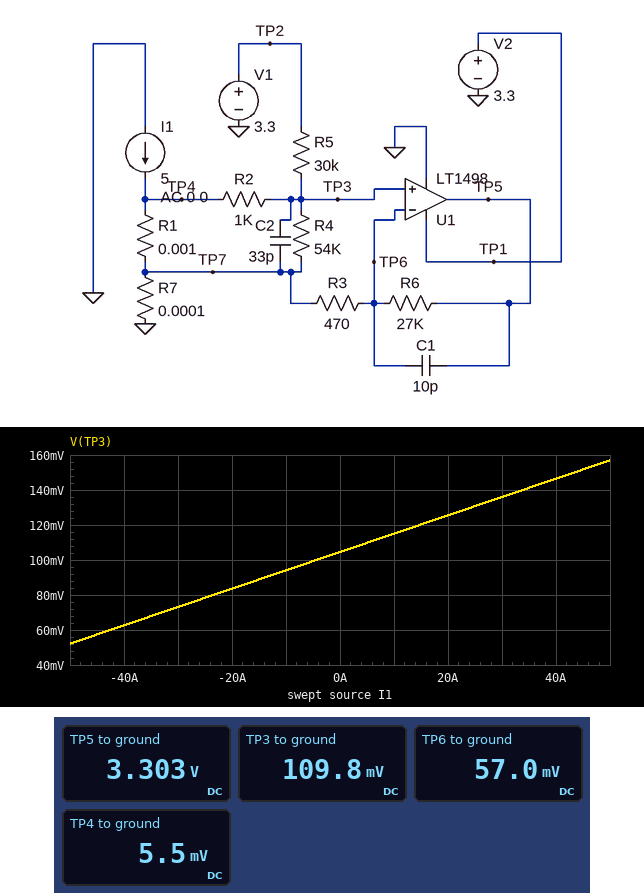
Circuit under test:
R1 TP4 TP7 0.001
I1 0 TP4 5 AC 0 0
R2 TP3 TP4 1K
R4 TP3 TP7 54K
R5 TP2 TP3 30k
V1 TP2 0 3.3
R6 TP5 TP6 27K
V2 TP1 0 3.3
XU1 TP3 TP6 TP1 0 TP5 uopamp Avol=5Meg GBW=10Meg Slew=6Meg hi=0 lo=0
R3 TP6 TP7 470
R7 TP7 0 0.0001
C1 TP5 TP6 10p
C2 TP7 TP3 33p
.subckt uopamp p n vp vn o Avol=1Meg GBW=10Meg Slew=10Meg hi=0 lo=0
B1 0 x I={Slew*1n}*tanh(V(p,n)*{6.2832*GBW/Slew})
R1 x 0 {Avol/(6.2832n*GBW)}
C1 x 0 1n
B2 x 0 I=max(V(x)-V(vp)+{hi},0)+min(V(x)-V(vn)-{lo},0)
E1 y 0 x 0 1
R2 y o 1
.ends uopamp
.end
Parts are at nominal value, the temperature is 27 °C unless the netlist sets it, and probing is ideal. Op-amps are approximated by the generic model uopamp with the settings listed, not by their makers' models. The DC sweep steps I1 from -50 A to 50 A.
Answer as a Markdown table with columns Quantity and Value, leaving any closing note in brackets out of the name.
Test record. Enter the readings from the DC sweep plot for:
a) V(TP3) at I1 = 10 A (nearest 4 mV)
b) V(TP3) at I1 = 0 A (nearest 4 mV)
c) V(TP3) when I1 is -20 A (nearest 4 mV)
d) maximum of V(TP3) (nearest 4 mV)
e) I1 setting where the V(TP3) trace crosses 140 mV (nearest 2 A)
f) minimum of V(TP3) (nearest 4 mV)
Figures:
| Quantity | Value |
|---|---|
| V(TP3) at I1 = 10 A | 116 mV |
| V(TP3) at I1 = 0 A | 104 mV |
| V(TP3) when I1 is -20 A | 84 mV |
| maximum of V(TP3) | 156 mV |
| I1 setting where the V(TP3) trace crosses 140 mV | 34 A |
| minimum of V(TP3) | 52 mV |
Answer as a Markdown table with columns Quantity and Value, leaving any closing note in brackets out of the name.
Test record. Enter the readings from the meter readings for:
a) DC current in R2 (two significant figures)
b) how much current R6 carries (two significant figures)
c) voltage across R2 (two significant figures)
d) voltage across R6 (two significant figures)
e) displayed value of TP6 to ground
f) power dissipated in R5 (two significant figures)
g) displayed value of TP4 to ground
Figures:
| Quantity | Value |
|---|---|
| DC current in R2 | 100 µA |
| how much current R6 carries | 120 µA |
| voltage across R2 | 100 mV |
| voltage across R6 | 3.2 V |
| displayed value of TP6 to ground | 57.0 mV |
| power dissipated in R5 | 340 µW |
| displayed value of TP4 to ground | 5.5 mV |
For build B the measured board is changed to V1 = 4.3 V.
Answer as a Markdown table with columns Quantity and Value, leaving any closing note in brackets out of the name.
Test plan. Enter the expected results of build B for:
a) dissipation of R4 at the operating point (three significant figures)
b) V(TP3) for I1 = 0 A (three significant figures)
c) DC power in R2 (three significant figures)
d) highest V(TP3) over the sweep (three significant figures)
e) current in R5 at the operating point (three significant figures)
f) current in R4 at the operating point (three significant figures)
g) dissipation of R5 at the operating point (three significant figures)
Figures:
| Quantity | Value |
|---|---|
| dissipation of R4 at the operating point | 368 nW |
| V(TP3) for I1 = 0 A | 136 mV |
| DC power in R2 | 18.5 µW |
| highest V(TP3) over the sweep | 189 mV |
| current in R5 at the operating point | 139 µA |
| current in R4 at the operating point | 2.61 µA |
| dissipation of R5 at the operating point | 576 µW |
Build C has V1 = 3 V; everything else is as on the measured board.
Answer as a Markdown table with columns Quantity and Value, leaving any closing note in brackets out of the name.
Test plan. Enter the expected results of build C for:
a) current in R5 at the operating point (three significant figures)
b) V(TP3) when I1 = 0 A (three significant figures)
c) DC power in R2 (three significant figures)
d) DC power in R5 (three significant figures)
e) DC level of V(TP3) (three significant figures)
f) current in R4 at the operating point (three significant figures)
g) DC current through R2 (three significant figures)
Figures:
| Quantity | Value |
|---|---|
| current in R5 at the operating point | 96.7 µA |
| V(TP3) when I1 = 0 A | 95.1 mV |
| DC power in R2 | 8.99 µW |
| DC power in R5 | 280 µW |
| DC level of V(TP3) | 100 mV |
| current in R4 at the operating point | 1.85 µA |
| DC current through R2 | 94.8 µA |
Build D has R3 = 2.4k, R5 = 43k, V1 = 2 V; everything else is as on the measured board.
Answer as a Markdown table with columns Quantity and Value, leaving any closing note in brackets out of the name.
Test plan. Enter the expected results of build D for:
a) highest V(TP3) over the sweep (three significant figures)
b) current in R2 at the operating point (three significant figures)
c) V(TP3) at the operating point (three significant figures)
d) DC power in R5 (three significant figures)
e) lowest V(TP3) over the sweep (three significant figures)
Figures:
| Quantity | Value |
|---|---|
| highest V(TP3) over the sweep | 97.5 mV |
| current in R2 at the operating point | 44.4 µA |
| V(TP3) at the operating point | 49.9 mV |
| DC power in R5 | 88.4 µW |
| lowest V(TP3) over the sweep | -8.24 mV |
